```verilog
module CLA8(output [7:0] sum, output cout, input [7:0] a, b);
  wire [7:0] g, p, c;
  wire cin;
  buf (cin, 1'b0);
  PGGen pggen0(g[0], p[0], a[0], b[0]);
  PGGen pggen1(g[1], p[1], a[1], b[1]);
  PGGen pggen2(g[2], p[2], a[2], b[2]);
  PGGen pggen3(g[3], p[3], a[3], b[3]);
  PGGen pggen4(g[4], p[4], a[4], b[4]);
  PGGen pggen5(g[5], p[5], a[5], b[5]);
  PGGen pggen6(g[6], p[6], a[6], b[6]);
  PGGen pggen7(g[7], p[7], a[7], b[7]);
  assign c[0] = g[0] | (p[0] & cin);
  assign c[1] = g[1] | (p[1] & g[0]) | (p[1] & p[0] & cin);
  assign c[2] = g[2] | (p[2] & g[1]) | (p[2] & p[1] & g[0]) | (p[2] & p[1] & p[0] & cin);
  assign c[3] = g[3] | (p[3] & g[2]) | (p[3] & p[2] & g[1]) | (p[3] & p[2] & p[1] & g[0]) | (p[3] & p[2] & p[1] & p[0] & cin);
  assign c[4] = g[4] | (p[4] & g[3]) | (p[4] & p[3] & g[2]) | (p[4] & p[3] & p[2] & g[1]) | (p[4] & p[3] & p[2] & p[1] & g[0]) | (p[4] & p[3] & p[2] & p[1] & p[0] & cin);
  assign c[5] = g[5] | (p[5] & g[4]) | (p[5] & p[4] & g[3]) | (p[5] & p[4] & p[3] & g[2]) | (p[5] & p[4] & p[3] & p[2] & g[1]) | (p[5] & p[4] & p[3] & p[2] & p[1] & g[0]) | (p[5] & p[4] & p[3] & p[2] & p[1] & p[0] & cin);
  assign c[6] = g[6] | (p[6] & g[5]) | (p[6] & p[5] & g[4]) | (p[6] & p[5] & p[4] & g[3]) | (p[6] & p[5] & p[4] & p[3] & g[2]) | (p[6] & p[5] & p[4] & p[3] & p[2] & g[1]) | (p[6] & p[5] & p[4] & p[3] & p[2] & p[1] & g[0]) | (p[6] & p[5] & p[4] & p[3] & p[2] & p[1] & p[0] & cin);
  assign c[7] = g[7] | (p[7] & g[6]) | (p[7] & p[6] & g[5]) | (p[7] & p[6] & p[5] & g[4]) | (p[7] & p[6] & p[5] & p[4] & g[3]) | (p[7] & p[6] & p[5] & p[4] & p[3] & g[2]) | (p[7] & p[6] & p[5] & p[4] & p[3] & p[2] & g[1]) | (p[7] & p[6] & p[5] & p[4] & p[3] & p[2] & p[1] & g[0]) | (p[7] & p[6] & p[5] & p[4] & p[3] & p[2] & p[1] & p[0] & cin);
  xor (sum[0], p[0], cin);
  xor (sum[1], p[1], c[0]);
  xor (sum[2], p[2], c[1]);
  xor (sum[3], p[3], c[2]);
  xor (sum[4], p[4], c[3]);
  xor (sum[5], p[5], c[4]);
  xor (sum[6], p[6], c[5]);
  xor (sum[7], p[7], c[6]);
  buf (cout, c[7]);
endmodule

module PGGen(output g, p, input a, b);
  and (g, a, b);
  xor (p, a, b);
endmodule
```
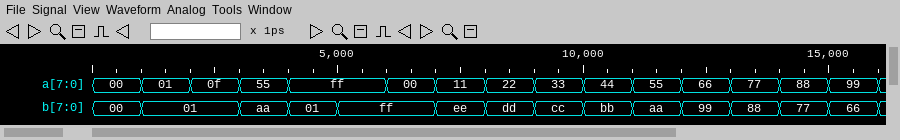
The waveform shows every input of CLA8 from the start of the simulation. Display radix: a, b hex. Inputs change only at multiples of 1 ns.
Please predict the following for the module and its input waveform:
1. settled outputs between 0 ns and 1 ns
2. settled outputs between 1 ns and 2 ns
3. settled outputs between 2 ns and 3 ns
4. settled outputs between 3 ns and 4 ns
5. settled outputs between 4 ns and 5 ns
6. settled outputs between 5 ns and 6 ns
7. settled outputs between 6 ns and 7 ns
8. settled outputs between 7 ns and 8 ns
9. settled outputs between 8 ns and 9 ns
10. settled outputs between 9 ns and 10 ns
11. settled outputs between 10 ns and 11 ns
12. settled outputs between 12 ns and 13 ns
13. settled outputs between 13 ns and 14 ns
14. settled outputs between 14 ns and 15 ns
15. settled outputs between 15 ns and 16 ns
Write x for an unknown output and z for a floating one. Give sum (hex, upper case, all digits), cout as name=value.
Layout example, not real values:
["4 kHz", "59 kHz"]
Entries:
["sum=00, cout=0", "sum=02, cout=0", "sum=10, cout=0", "sum=FF, cout=0", "sum=00, cout=1", "sum=FE, cout=1", "sum=FF, cout=0", "sum=FF, cout=0", "sum=FF, cout=0", "sum=FF, cout=0", "sum=FF, cout=0", "sum=FF, cout=0", "sum=FF, cout=0", "sum=FF, cout=0", "sum=FF, cout=0"]
